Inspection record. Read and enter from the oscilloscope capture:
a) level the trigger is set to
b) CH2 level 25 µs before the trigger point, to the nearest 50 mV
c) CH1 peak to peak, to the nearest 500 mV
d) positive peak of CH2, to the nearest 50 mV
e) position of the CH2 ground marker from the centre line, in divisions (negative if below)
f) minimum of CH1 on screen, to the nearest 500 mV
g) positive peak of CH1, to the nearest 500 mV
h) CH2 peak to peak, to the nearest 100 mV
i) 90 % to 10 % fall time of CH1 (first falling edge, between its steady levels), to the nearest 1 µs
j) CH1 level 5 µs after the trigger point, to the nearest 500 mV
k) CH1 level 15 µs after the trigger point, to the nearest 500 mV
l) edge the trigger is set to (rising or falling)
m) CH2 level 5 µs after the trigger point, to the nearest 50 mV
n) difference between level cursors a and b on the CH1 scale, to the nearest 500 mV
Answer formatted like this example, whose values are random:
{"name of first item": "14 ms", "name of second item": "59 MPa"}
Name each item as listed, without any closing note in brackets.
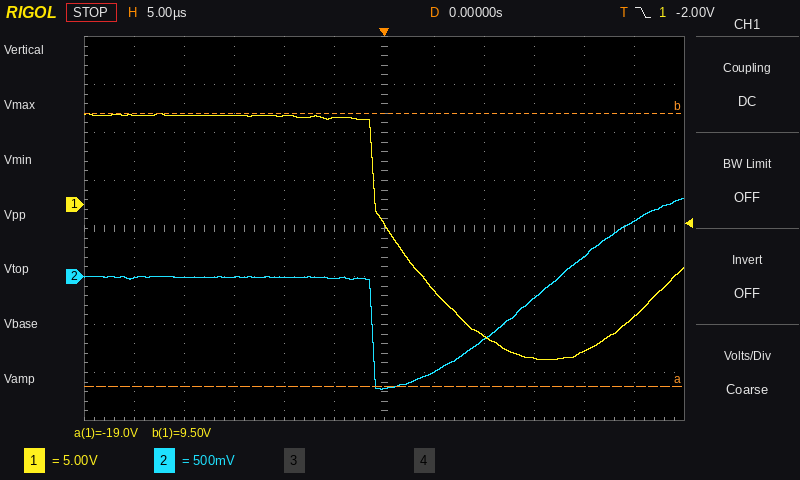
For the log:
{"level the trigger is set to": "-2.00 V", "CH2 level 25 µs before the trigger point, to the nearest 50 mV": "0 mV", "CH1 peak to peak, to the nearest 500 mV": "25.5 V", "positive peak of CH2, to the nearest 50 mV": "800 mV", "position of the CH2 ground marker from the centre line, in divisions": "-1.0 div", "minimum of CH1 on screen, to the nearest 500 mV": "-16.0 V", "positive peak of CH1, to the nearest 500 mV": "9.5 V", "CH2 peak to peak, to the nearest 100 mV": "2.00 V", "90 % to 10 % fall time of CH1 (first falling edge, between its steady levels), to the nearest 1 µs": "11 µs", "CH1 level 5 µs after the trigger point, to the nearest 500 mV": "-9.0 V", "CH1 level 15 µs after the trigger point, to the nearest 500 mV": "-16.0 V", "edge the trigger is set to": "falling", "CH2 level 5 µs after the trigger point, to the nearest 50 mV": "-1.00 V", "difference between level cursors a and b on the CH1 scale, to the nearest 500 mV": "28.5 V"}
